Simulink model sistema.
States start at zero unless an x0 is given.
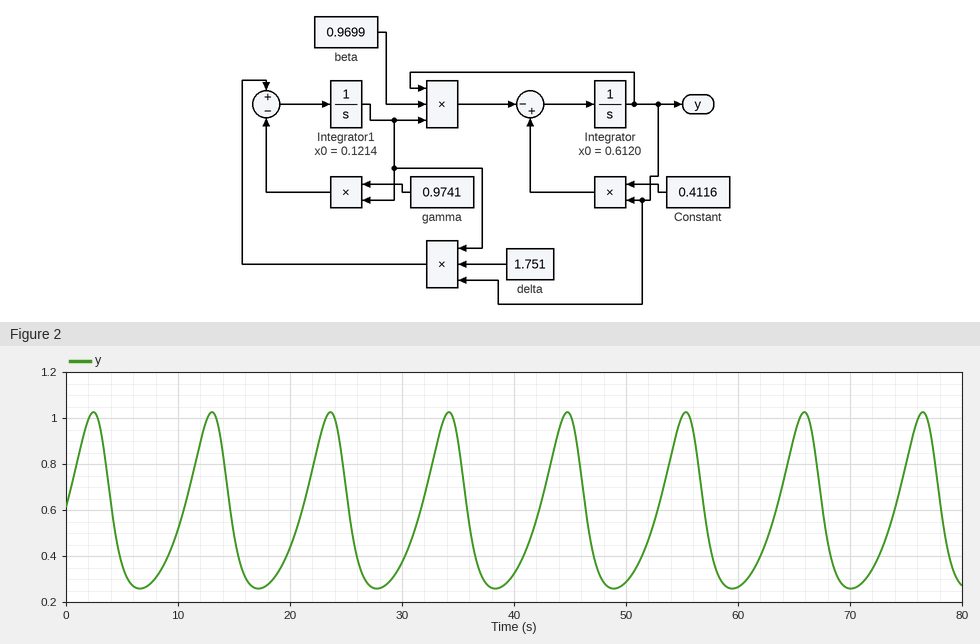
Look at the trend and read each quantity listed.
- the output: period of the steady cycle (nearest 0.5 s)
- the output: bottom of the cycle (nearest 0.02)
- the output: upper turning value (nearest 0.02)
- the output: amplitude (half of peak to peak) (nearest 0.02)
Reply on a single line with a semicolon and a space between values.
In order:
10.5 s; 0.26; 1.02; 0.38
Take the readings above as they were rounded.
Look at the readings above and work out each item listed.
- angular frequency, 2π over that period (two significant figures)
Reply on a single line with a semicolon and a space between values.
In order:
0.60 rad/s
